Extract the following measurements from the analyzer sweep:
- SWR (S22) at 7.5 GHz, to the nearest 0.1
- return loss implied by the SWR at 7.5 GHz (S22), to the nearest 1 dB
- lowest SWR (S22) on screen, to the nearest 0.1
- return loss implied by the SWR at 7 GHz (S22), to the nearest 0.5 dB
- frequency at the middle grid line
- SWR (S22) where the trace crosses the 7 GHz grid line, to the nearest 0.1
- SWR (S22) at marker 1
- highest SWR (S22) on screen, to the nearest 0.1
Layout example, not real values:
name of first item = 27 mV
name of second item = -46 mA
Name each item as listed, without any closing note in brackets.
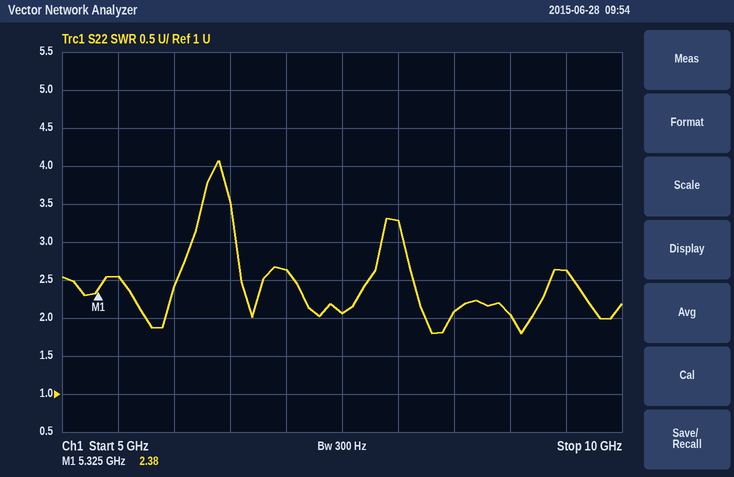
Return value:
SWR (S22) at 7.5 GHz, to the nearest 0.1 = 2.1
return loss implied by the SWR at 7.5 GHz (S22), to the nearest 1 dB = 9 dB
lowest SWR (S22) on screen, to the nearest 0.1 = 1.8
return loss implied by the SWR at 7 GHz (S22), to the nearest 0.5 dB = 7.0 dB
frequency at the middle grid line = 7.5 GHz
SWR (S22) where the trace crosses the 7 GHz grid line, to the nearest 0.1 = 2.6
SWR (S22) at marker 1 = 2.38
highest SWR (S22) on screen, to the nearest 0.1 = 4.1
